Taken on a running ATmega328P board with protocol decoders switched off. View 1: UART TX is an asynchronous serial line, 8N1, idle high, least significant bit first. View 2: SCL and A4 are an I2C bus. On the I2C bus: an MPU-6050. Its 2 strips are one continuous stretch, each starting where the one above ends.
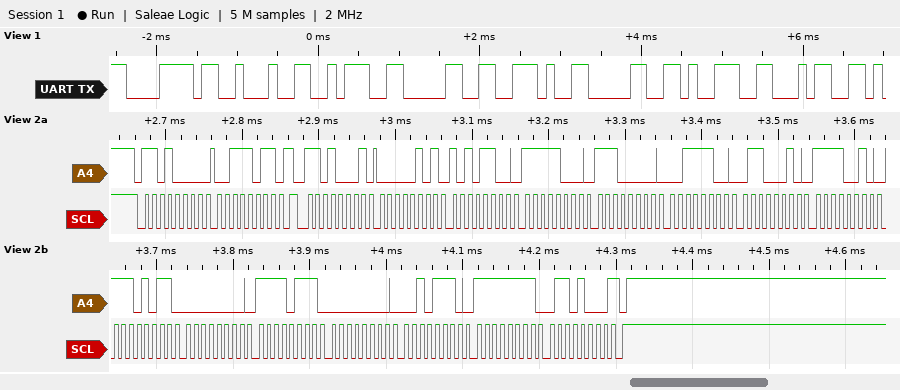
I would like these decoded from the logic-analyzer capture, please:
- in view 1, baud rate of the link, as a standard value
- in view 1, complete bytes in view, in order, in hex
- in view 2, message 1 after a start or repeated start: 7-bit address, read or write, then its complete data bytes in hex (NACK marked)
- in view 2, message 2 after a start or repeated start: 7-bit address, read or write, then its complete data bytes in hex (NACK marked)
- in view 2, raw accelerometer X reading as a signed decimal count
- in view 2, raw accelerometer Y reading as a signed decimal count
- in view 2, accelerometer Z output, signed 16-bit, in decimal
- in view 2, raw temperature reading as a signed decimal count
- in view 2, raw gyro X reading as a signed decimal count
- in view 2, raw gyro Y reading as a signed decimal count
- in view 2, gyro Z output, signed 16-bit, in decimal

9600 baud
78 22 3A 30 2E 30 39 34
0x68 write: 3B
0x68 read: 05 AC F8 E0 3C 62 F2 EB 00 F7 00 2E FF 68 NACK
1452
-1824
15458
-3349
247
46
-152
